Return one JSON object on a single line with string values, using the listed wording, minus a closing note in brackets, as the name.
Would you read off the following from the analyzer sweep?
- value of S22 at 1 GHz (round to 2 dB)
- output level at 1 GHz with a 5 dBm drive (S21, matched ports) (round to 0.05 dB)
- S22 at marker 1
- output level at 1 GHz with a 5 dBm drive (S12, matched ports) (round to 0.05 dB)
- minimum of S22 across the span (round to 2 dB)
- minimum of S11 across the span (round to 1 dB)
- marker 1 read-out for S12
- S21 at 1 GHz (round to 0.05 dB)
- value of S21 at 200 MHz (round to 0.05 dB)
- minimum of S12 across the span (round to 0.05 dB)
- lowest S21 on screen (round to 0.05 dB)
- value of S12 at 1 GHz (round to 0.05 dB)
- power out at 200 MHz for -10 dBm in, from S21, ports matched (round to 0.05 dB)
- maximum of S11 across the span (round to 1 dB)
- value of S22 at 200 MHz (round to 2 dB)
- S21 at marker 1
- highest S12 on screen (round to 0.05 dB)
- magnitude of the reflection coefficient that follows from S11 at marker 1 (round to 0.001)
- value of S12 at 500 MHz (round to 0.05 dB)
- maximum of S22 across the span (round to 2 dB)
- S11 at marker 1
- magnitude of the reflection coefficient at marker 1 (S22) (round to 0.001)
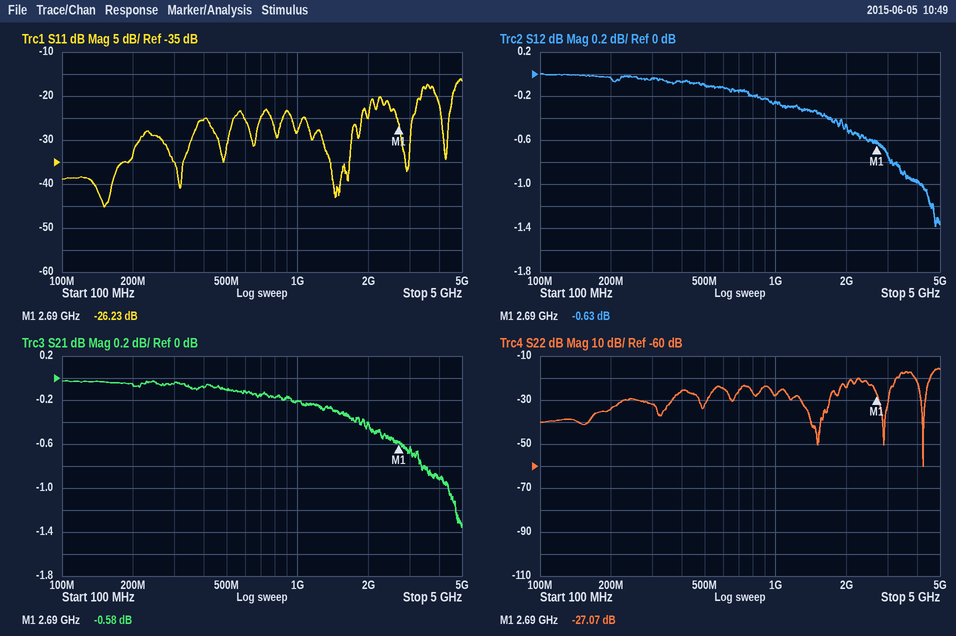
{"value of S22 at 1 GHz": "-28 dB", "output level at 1 GHz with a 5 dBm drive (S21, matched ports)": "4.80 dBm", "S22 at marker 1": "-27.07 dB", "output level at 1 GHz with a 5 dBm drive (S12, matched ports)": "4.75 dBm", "minimum of S22 across the span": "-60 dB", "minimum of S11 across the span": "-45 dB", "marker 1 read-out for S12": "-0.63 dB", "S21 at 1 GHz": "-0.20 dB", "value of S21 at 200 MHz": "-0.05 dB", "minimum of S12 across the span": "-1.40 dB", "lowest S21 on screen": "-1.35 dB", "value of S12 at 1 GHz": "-0.25 dB", "power out at 200 MHz for -10 dBm in, from S21, ports matched": "-10.05 dBm", "maximum of S11 across the span": "-16 dB", "value of S22 at 200 MHz": "-34 dB", "S21 at marker 1": "-0.58 dB", "highest S12 on screen": "0.00 dB", "magnitude of the reflection coefficient that follows from S11 at marker 1": "0.049", "value of S12 at 500 MHz": "-0.10 dB", "maximum of S22 across the span": "-16 dB", "S11 at marker 1": "-26.23 dB", "magnitude of the reflection coefficient at marker 1 (S22)": "0.044"}
